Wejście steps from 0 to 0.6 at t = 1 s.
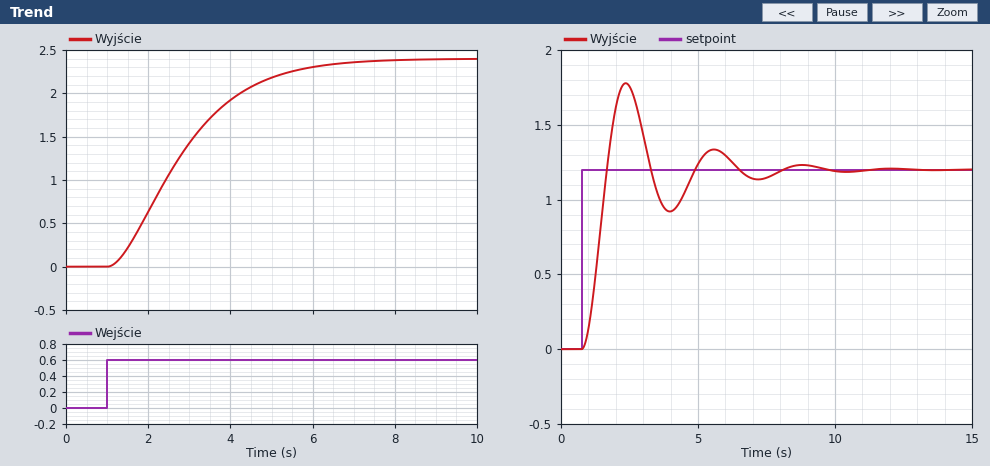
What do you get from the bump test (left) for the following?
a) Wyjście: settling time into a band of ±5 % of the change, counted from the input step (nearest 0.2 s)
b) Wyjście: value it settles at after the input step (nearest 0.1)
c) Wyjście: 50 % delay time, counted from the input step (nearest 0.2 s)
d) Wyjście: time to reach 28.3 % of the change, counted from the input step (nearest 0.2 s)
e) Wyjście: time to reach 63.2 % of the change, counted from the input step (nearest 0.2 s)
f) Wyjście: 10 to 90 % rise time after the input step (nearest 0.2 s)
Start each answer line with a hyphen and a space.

- 4.8 s
- 2.4
- 1.6 s
- 1.0 s
- 2.2 s
- 3.4 s
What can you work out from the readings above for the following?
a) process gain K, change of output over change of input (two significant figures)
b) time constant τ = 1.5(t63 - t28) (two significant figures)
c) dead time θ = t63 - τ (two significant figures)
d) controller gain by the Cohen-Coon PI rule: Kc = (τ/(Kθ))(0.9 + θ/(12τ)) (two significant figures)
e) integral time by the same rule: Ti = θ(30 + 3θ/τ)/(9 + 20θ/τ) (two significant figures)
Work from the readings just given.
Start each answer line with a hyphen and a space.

- 4.0
- 1.8 s
- 0.40 s
- 1.0
- 0.91 s
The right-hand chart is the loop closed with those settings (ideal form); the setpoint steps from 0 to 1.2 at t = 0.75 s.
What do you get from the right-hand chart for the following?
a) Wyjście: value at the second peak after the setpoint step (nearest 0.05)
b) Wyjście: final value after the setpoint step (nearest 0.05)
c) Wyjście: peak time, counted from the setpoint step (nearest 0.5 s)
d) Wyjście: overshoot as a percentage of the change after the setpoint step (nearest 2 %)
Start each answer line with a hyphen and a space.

- 1.35
- 1.20
- 1.5 s
- 48 %
